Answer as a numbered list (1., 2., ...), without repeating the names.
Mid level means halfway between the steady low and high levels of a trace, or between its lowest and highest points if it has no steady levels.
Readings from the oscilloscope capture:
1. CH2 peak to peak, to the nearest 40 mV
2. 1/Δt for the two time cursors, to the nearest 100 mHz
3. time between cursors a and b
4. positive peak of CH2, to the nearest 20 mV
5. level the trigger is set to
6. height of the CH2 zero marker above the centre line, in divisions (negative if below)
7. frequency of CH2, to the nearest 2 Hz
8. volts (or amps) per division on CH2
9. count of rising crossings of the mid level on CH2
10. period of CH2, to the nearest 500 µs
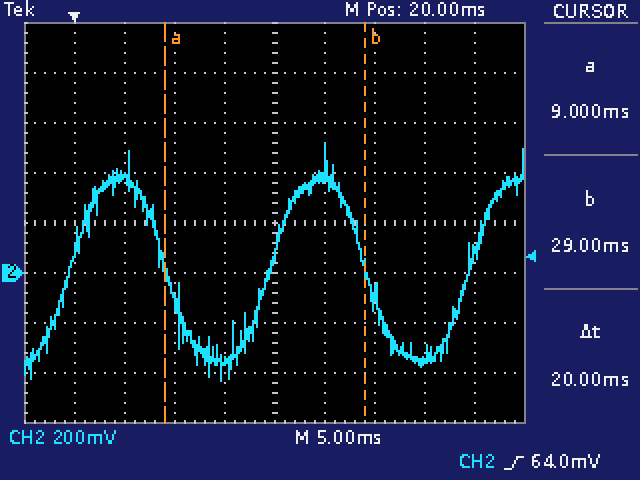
1. 960 mV
2. 50.0 Hz
3. 20 ms
4. 520 mV
5. 64.0 mV
6. -1.0 div
7. 50 Hz
8. 200 mV
9. 3
10. 20.0 ms
